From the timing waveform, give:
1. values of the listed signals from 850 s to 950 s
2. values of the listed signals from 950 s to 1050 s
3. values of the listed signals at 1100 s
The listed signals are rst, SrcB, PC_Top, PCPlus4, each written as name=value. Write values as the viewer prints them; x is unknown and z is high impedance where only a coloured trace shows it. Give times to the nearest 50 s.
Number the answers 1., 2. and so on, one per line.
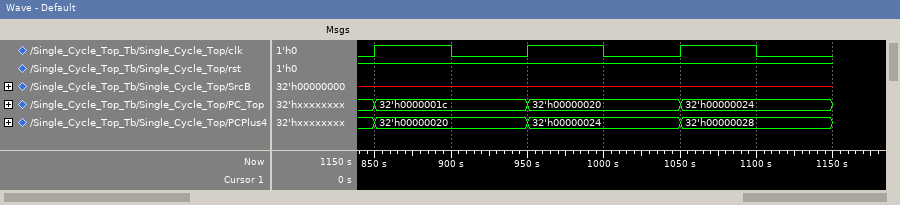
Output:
1. rst=1, SrcB=x, PC_Top=32'h0000001c, PCPlus4=32'h00000020
2. rst=1, SrcB=x, PC_Top=32'h00000020, PCPlus4=32'h00000024
3. rst=1, SrcB=x, PC_Top=32'h00000024, PCPlus4=32'h00000028
